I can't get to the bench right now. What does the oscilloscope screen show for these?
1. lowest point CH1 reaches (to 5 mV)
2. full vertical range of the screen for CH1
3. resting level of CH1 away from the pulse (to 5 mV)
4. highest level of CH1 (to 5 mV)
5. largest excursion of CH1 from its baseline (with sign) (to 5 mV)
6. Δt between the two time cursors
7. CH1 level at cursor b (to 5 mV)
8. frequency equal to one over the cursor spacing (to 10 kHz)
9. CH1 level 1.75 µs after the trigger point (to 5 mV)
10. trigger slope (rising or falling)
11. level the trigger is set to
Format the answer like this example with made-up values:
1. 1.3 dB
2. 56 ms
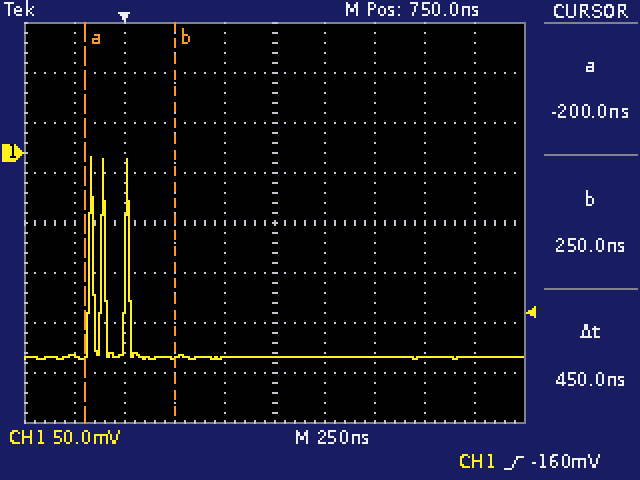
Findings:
1. -205 mV
2. 400 mV
3. -205 mV
4. -5 mV
5. +200 mV
6. 450 ns
7. -205 mV
8. 2.22 MHz
9. -205 mV
10. rising
11. -160 mV
